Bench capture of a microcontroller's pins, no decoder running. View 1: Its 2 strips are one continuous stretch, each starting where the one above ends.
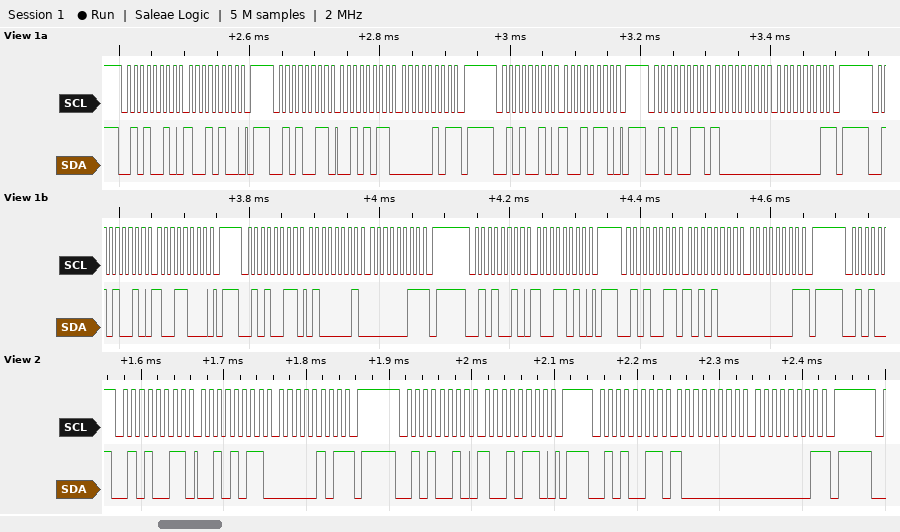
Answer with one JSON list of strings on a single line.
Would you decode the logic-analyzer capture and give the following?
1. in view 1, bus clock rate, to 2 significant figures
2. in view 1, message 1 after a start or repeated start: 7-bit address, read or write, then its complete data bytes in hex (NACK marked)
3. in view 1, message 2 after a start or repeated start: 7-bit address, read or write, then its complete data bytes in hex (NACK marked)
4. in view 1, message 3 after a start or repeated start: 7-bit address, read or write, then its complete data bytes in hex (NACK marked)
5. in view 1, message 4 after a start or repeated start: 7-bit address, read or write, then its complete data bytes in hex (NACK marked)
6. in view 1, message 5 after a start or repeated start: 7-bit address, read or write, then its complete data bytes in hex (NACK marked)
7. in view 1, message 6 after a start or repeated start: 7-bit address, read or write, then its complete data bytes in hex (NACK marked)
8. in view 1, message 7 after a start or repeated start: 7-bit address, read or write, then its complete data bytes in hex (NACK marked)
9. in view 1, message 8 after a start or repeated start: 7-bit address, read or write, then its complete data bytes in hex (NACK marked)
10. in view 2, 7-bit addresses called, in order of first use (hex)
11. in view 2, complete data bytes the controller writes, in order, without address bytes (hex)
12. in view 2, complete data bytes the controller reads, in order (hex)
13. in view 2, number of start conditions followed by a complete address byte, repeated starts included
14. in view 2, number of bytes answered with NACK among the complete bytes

["100 kHz", "0x29 write: 94", "0x29 read: 2B 05 NACK", "0x29 write: 96", "0x29 read: 80 01 NACK", "0x29 write: 98", "0x29 read: 41 03 NACK", "0x29 write: 9A", "0x29 read: A8 01 NACK", "0x29", "96", "2B 05 80 01", "3", "2"]
